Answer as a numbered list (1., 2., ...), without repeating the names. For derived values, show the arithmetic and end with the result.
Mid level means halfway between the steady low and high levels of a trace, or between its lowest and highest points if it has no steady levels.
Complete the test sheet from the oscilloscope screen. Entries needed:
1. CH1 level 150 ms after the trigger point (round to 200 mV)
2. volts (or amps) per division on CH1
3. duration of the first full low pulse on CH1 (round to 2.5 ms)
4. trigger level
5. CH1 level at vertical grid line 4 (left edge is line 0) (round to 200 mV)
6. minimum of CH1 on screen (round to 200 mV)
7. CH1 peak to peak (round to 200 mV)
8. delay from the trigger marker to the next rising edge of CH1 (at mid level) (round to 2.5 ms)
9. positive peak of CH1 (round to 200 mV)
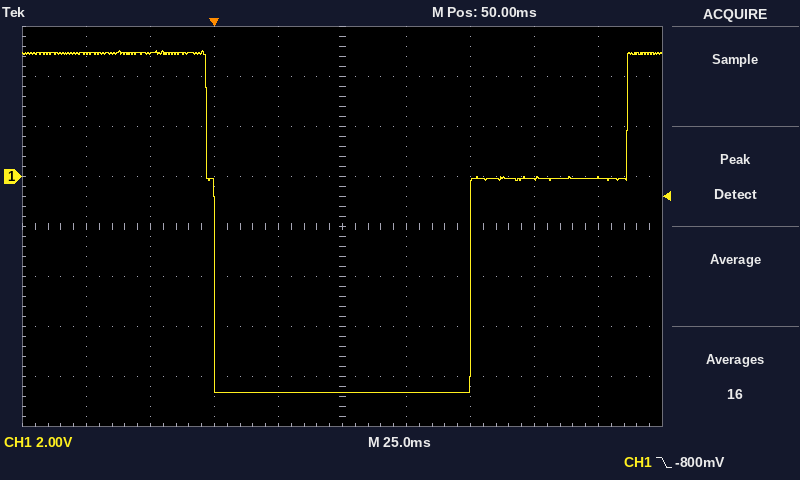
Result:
1. 0.0 V
2. 2 V
3. 100.0 ms
4. -800 mV
5. -8.6 V
6. -8.6 V
7. 5.0 V − (-8.6 V) = 13.6 V
8. 100.0 ms
9. 5.0 V
